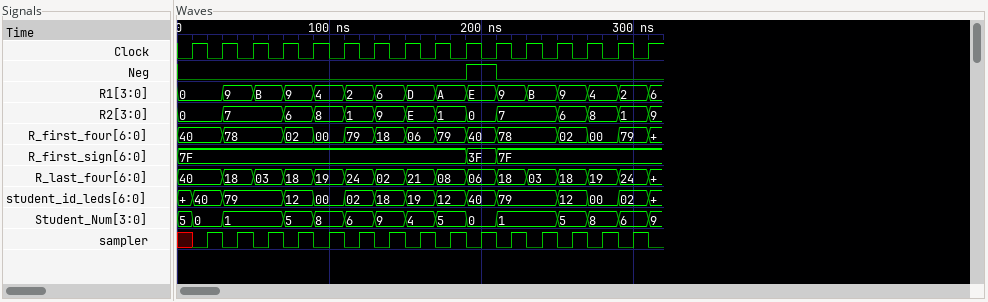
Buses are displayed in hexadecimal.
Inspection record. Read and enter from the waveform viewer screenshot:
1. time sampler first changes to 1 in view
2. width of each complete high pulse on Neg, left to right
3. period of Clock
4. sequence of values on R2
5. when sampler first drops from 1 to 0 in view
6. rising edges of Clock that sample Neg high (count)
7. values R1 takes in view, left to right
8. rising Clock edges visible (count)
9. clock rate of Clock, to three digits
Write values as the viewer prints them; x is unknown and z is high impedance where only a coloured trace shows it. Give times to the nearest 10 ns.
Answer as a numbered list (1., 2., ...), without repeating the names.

1. 20 ns
2. 20 ns
3. 20 ns
4. 0, 7, 6, 8, 1, 9, E, 1, 0, 7, 6, 8, 1, 9
5. 30 ns
6. 1
7. 0, 9, B, 9, 4, 2, 6, D, A, E, 9, B, 9, 4, 2, 6
8. 16
9. 50.0 MHz
